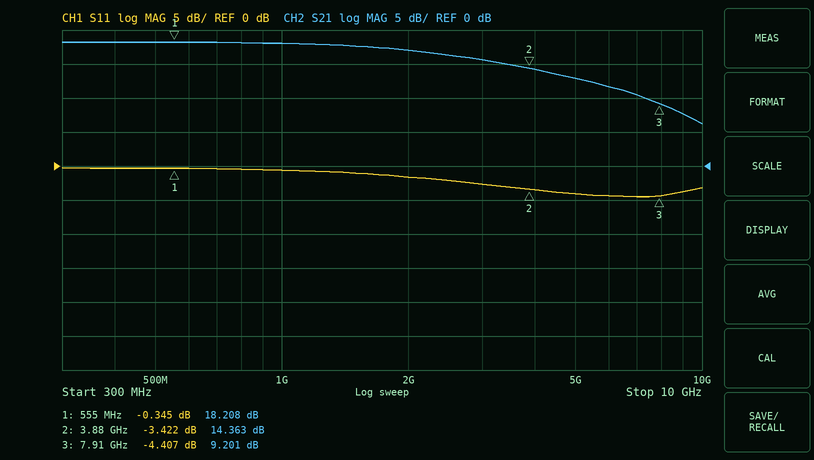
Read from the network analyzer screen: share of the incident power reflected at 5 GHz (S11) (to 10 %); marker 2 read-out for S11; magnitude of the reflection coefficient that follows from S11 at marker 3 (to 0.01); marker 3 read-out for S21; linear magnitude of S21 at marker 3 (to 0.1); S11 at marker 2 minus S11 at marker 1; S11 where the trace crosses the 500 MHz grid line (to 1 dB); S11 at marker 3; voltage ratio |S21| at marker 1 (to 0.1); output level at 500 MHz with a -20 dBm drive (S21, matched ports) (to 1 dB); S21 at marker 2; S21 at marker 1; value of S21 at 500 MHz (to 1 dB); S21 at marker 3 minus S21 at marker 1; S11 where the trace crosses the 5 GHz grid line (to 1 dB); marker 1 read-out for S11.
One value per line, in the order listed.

40 %
-3.422 dB
0.60
9.201 dB
2.9
-3.077 dB
0 dB
-4.407 dB
8.1
-2 dBm
14.363 dB
18.208 dB
18 dB
-9.007 dB
-4 dB
-0.345 dB
